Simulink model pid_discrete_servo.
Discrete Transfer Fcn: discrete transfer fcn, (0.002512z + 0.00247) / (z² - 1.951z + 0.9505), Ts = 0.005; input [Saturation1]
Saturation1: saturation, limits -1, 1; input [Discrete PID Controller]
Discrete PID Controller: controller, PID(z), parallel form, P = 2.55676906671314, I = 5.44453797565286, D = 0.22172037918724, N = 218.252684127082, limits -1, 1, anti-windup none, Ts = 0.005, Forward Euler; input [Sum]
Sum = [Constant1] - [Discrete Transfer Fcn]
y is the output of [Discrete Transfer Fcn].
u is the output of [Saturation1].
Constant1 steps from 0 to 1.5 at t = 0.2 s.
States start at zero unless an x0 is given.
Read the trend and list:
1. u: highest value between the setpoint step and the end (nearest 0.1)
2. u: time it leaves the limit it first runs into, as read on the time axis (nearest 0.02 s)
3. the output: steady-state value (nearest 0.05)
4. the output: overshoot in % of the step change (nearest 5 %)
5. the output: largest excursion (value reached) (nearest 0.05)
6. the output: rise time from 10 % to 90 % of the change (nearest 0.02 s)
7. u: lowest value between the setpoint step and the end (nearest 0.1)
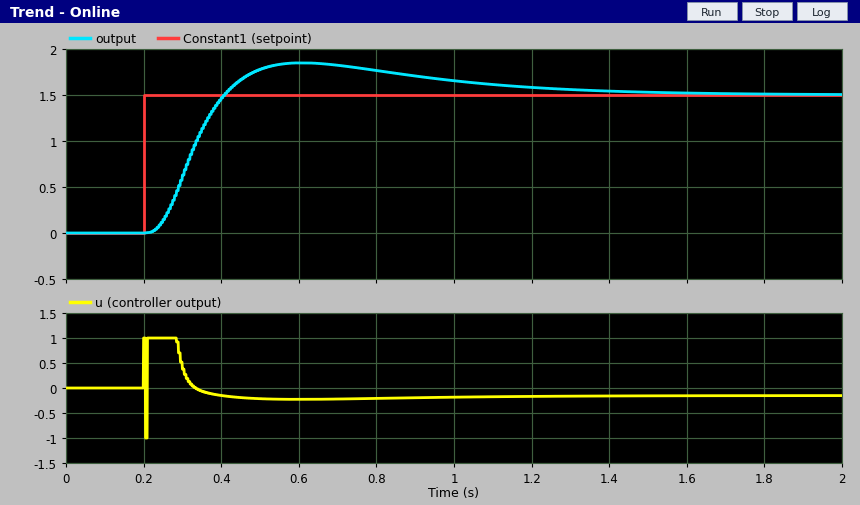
1.0
0.28 s
1.50
25 %
1.85
0.12 s
-1.0
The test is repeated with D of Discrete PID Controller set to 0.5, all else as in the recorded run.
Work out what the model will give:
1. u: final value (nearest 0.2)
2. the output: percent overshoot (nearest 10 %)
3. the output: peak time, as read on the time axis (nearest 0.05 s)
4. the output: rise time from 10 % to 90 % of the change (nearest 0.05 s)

-0.2
30 %
0.90 s
0.25 s
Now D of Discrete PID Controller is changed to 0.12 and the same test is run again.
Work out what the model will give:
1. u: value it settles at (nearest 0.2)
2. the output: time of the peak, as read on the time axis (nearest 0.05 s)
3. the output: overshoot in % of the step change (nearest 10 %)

-0.2
0.45 s
30 %
